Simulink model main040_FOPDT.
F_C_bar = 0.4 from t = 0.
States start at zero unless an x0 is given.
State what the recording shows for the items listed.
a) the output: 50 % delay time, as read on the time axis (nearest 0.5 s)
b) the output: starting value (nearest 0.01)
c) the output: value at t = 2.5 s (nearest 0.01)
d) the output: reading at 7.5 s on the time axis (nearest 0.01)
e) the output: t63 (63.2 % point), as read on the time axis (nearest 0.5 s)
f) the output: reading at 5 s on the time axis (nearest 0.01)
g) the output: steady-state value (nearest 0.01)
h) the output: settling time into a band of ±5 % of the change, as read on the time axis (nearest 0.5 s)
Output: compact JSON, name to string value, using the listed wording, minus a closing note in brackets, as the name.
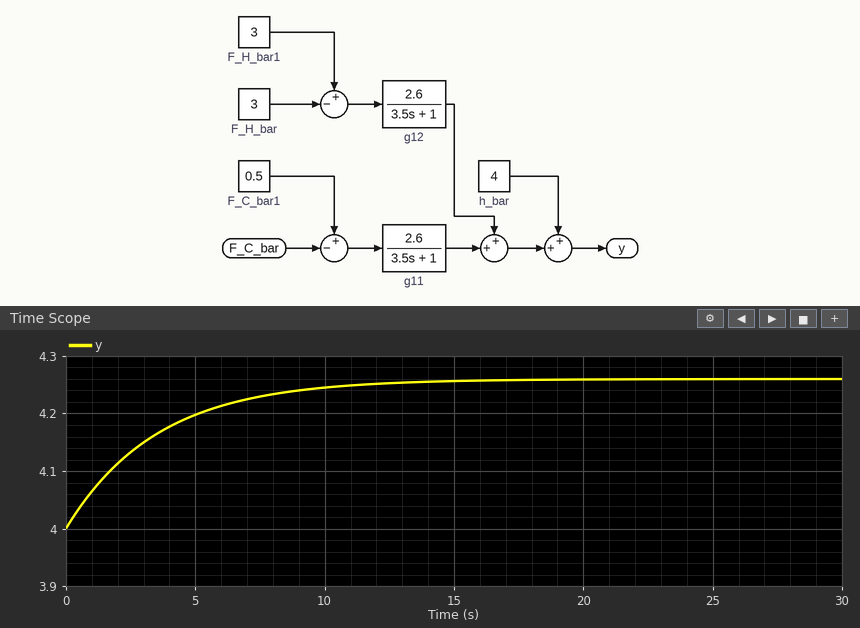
{"the output: 50 % delay time, as read on the time axis": "2.5 s", "the output: starting value": "4.00", "the output: value at t = 2.5 s": "4.13", "the output: reading at 7.5 s on the time axis": "4.23", "the output: t63 (63.2 % point), as read on the time axis": "3.5 s", "the output: reading at 5 s on the time axis": "4.20", "the output: steady-state value": "4.26", "the output: settling time into a band of ±5 % of the change, as read on the time axis": "10.5 s"}
